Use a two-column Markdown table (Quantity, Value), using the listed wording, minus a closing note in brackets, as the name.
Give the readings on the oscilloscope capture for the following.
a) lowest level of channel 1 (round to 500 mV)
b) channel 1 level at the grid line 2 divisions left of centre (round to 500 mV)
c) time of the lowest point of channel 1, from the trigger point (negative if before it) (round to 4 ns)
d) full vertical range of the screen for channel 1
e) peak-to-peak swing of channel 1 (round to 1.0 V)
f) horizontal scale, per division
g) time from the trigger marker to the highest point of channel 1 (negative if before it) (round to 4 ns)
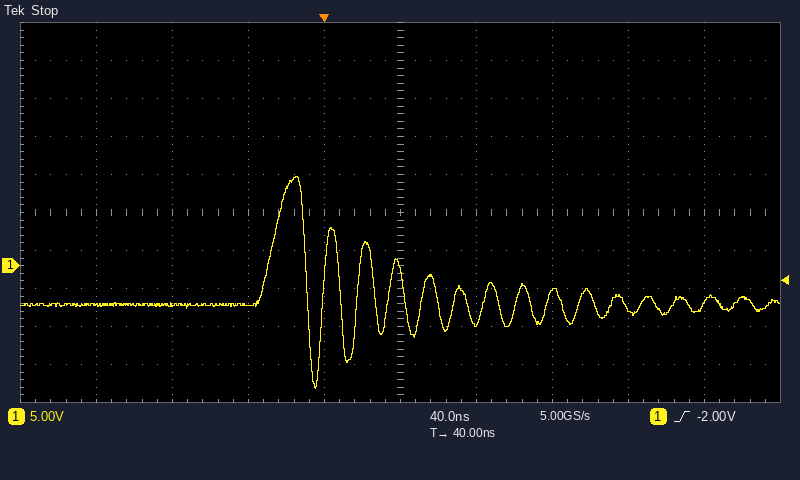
| Quantity | Value |
|---|---|
| lowest level of channel 1 | -16.0 V |
| channel 1 level at the grid line 2 divisions left of centre | -5.0 V |
| time of the lowest point of channel 1, from the trigger point (negative if before it) | -4 ns |
| full vertical range of the screen for channel 1 | 50 V |
| peak-to-peak swing of channel 1 | 28.0 V |
| horizontal scale, per division | 40 ns |
| time from the trigger marker to the highest point of channel 1 (negative if before it) | -16 ns |
